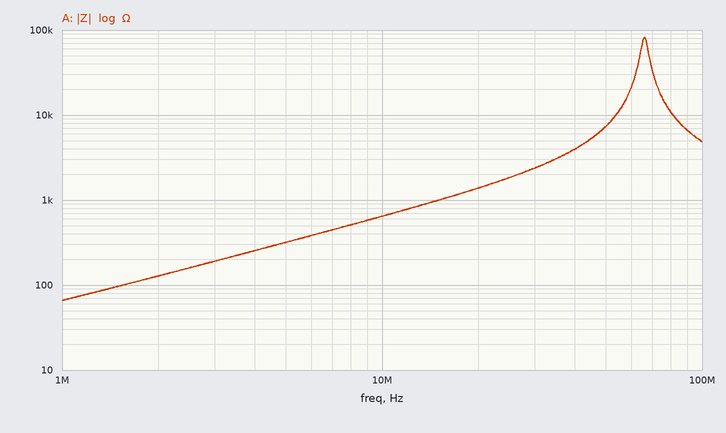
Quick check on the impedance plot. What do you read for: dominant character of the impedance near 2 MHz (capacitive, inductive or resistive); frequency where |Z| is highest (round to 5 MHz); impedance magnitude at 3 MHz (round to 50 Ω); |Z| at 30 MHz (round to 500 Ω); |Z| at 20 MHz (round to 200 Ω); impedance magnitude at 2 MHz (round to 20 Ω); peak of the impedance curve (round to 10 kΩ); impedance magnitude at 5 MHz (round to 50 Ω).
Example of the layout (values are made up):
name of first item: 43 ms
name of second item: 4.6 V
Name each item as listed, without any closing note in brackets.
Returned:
dominant character of the impedance near 2 MHz: inductive
frequency where |Z| is highest: 65 MHz
impedance magnitude at 3 MHz: 200 Ω
|Z| at 30 MHz: 2.5 kΩ
|Z| at 20 MHz: 1.4 kΩ
impedance magnitude at 2 MHz: 120 Ω
peak of the impedance curve: 80 kΩ
impedance magnitude at 5 MHz: 300 Ω
